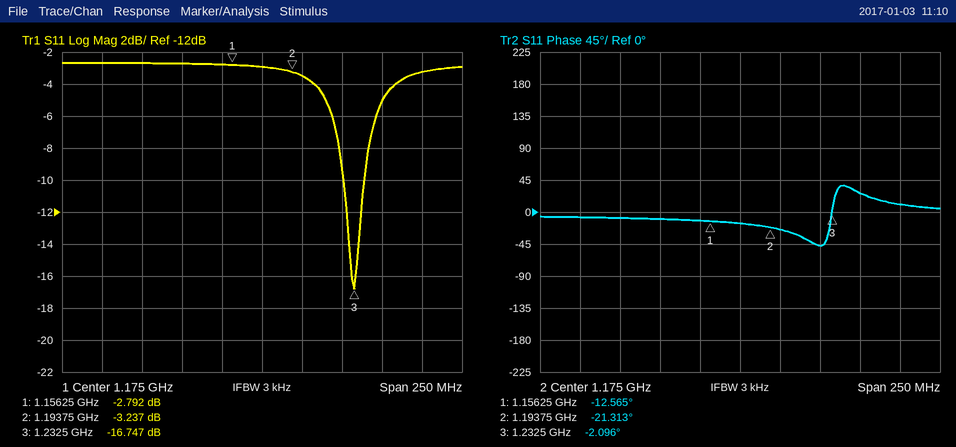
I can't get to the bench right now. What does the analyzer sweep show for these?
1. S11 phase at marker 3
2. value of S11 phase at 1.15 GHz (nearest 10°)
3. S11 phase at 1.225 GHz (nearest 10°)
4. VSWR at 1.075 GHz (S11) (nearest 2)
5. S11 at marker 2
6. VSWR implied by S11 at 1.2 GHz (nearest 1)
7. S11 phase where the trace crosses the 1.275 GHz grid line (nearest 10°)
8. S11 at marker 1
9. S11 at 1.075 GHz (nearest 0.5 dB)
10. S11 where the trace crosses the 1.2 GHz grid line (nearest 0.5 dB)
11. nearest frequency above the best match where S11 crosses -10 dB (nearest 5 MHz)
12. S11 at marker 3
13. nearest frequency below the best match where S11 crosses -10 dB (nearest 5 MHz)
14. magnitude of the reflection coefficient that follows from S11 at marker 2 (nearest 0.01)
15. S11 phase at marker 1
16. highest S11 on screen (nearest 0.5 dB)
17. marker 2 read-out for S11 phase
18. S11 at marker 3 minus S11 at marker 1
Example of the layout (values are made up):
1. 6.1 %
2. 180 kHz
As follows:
1. -2.096°
2. -10°
3. -50°
4. 6
5. -3.237 dB
6. 5
7. 10°
8. -2.792 dB
9. -2.5 dB
10. -3.5 dB
11. 1.240 GHz
12. -16.747 dB
13. 1.225 GHz
14. 0.69
15. -12.565°
16. -2.5 dB
17. -21.313°
18. -13.955 dB
